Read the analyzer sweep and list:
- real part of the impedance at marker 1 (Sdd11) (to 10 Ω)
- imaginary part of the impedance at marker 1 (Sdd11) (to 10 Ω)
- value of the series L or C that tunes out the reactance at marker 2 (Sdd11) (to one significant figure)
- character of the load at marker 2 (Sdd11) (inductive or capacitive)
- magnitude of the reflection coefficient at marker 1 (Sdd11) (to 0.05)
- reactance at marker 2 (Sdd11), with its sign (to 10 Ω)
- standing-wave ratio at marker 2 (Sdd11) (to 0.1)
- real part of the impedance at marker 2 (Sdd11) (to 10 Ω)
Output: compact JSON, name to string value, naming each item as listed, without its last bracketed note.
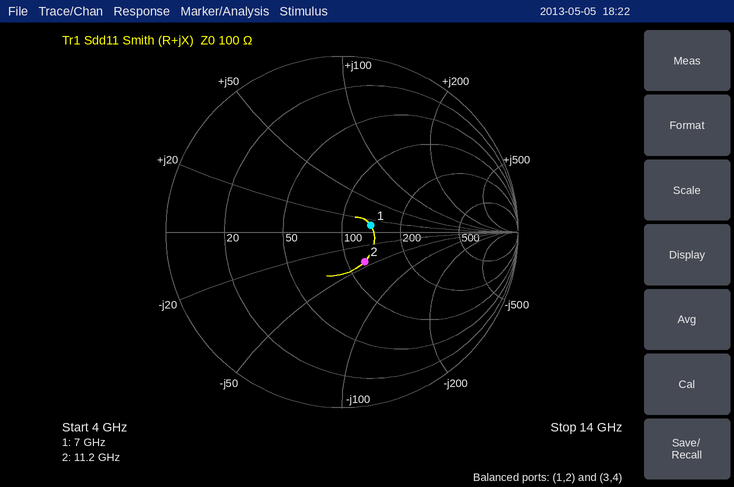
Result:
{"real part of the impedance at marker 1 (Sdd11)": "140 Ω", "imaginary part of the impedance at marker 1 (Sdd11)": "+10 Ω", "value of the series L or C that tunes out the reactance at marker 2 (Sdd11)": "600 pH", "character of the load at marker 2 (Sdd11)": "capacitive", "magnitude of the reflection coefficient at marker 1 (Sdd11)": "0.15", "reactance at marker 2 (Sdd11), with its sign": "-40 Ω", "standing-wave ratio at marker 2 (Sdd11)": "1.5", "real part of the impedance at marker 2 (Sdd11)": "120 Ω"}
